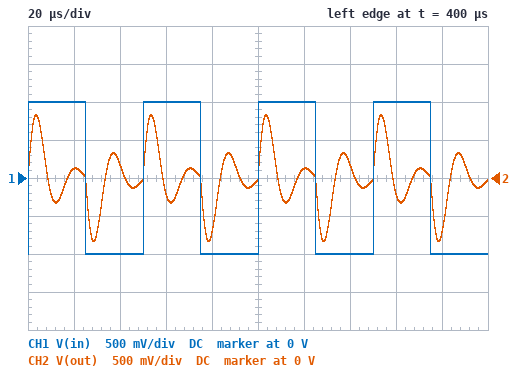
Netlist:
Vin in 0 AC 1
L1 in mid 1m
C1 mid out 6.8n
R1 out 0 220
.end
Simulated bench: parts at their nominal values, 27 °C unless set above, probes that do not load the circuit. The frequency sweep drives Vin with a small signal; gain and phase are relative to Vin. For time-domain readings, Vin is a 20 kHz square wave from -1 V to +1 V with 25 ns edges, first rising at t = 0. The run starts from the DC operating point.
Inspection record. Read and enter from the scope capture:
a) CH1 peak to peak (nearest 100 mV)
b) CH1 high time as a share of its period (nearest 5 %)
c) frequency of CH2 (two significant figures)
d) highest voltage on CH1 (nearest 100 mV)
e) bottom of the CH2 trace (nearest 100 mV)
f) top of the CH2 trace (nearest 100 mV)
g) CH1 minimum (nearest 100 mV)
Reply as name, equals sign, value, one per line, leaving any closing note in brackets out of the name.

CH1 peak to peak = 2.0 V
CH1 high time as a share of its period = 50 %
frequency of CH2 = 20 kHz
highest voltage on CH1 = 1.0 V
bottom of the CH2 trace = -800 mV
top of the CH2 trace = 800 mV
CH1 minimum = -1.0 V
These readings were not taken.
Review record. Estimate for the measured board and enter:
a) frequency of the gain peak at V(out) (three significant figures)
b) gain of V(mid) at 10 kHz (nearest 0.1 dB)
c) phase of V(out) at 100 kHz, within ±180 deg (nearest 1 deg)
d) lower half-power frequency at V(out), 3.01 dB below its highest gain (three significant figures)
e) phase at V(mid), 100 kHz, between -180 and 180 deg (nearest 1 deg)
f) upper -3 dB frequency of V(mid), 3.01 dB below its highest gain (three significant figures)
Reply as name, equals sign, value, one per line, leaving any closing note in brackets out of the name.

frequency of the gain peak at V(out) = 61.0 kHz
gain of V(mid) at 10 kHz = 0.2 dB
phase of V(out) at 100 kHz, within ±180 deg = -61 deg
lower half-power frequency at V(out), 3.01 dB below its highest gain = 46.0 kHz
phase at V(mid), 100 kHz, between -180 and 180 deg = -108 deg
upper -3 dB frequency of V(mid), 3.01 dB below its highest gain = 73.9 kHz
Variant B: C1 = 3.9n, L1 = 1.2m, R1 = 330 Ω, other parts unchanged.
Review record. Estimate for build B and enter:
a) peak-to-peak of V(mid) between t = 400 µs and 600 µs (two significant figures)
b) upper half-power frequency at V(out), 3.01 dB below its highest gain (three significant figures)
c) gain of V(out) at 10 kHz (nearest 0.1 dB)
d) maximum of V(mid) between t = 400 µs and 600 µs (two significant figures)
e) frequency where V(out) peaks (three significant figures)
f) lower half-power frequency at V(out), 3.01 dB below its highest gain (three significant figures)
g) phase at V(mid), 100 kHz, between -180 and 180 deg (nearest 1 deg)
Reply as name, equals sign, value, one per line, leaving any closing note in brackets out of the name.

peak-to-peak of V(mid) between t = 400 µs and 600 µs = 3.8 V
upper half-power frequency at V(out), 3.01 dB below its highest gain = 98.6 kHz
gain of V(out) at 10 kHz = -21.7 dB
maximum of V(mid) between t = 400 µs and 600 µs = 1.9 V
frequency where V(out) peaks = 73.6 kHz
lower half-power frequency at V(out), 3.01 dB below its highest gain = 54.9 kHz
phase at V(mid), 100 kHz, between -180 and 180 deg = -97 deg
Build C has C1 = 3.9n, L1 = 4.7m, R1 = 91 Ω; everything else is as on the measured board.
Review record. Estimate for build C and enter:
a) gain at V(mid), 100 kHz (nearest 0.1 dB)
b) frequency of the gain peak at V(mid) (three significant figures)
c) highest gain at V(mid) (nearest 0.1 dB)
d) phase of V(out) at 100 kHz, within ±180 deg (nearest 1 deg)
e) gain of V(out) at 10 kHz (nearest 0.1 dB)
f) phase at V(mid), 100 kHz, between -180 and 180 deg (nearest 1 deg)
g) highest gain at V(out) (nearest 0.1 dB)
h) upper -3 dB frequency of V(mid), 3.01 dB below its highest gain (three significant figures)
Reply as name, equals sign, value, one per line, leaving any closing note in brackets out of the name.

gain at V(mid), 100 kHz = -15.7 dB
frequency of the gain peak at V(mid) = 37.1 kHz
highest gain at V(mid) = 21.7 dB
phase of V(out) at 100 kHz, within ±180 deg = -88 deg
gain of V(out) at 10 kHz = -32.4 dB
phase at V(mid), 100 kHz, between -180 and 180 deg = -165 deg
highest gain at V(out) = 0 dB
upper -3 dB frequency of V(mid), 3.01 dB below its highest gain = 38.6 kHz
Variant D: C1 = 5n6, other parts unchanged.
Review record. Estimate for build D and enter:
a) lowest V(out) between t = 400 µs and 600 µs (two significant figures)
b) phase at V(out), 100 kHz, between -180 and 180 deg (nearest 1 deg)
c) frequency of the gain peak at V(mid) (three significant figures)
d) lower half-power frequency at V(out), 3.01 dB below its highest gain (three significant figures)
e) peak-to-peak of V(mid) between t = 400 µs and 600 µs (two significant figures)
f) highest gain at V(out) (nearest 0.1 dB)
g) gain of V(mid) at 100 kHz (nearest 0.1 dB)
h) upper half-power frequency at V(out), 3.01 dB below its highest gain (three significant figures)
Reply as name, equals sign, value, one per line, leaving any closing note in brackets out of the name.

lowest V(out) between t = 400 µs and 600 µs = -780 mV
phase at V(out), 100 kHz, between -180 and 180 deg = -57 deg
frequency of the gain peak at V(mid) = 63.5 kHz
lower half-power frequency at V(out), 3.01 dB below its highest gain = 52.0 kHz
peak-to-peak of V(mid) between t = 400 µs and 600 µs = 4.1 V
highest gain at V(out) = 0 dB
gain of V(mid) at 100 kHz = -1.1 dB
upper half-power frequency at V(out), 3.01 dB below its highest gain = 87.0 kHz
